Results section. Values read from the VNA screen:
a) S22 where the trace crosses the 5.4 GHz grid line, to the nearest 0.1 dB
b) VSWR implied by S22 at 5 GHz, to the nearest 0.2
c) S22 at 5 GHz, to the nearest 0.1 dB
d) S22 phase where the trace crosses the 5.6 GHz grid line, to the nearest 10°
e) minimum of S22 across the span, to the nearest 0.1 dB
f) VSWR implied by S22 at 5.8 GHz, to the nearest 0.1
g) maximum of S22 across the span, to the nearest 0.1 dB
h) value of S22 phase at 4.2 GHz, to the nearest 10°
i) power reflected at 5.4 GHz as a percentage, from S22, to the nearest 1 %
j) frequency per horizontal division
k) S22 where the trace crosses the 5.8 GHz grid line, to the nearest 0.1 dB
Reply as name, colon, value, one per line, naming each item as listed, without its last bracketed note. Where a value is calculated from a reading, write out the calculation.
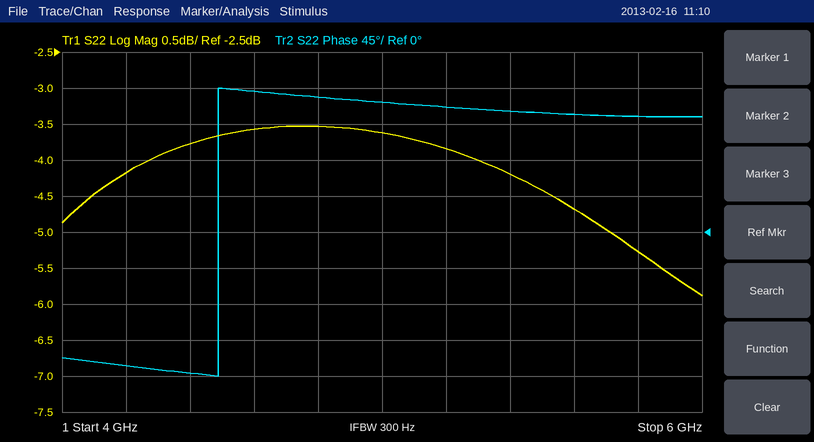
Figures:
S22 where the trace crosses the 5.4 GHz grid line, to the nearest 0.1 dB: -4.2 dB
VSWR implied by S22 at 5 GHz, to the nearest 0.2: |Γ| = 10^(-3.6/20) = 0.6607; VSWR = (1 + 0.6607)/(1 − 0.6607) ≈ 4.89, so 4.8 to the nearest 0.2
S22 at 5 GHz, to the nearest 0.1 dB: -3.6 dB
S22 phase where the trace crosses the 5.6 GHz grid line, to the nearest 10°: 150°
minimum of S22 across the span, to the nearest 0.1 dB: -5.9 dB
VSWR implied by S22 at 5.8 GHz, to the nearest 0.1: |Γ| = 10^(-5.3/20) = 0.5433; VSWR = (1 + 0.5433)/(1 − 0.5433) ≈ 3.4
maximum of S22 across the span, to the nearest 0.1 dB: -3.5 dB
value of S22 phase at 4.2 GHz, to the nearest 10°: -170°
power reflected at 5.4 GHz as a percentage, from S22, to the nearest 1 %: 10^(-4.2/10) ≈ 38 %
frequency per horizontal division: 200 MHz
S22 where the trace crosses the 5.8 GHz grid line, to the nearest 0.1 dB: -5.3 dB
